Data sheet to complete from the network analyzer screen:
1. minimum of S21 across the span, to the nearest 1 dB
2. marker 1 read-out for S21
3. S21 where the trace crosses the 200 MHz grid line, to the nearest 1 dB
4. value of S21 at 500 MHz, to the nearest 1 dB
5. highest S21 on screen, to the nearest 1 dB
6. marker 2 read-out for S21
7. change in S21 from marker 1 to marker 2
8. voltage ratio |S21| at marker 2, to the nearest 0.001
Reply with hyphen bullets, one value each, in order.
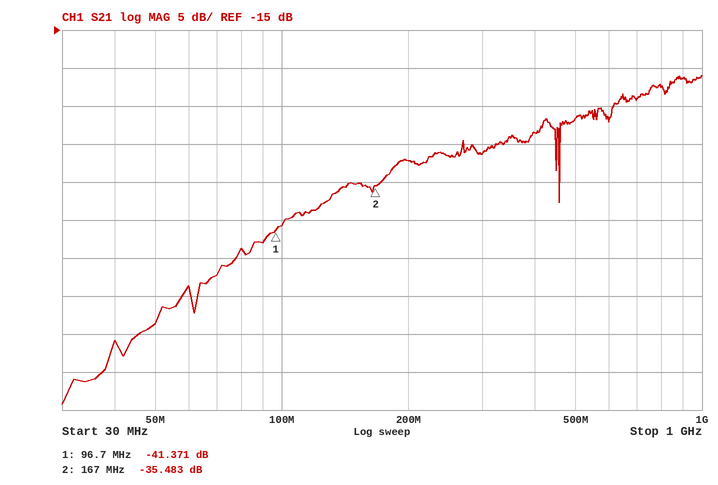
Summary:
- -64 dB
- -41.371 dB
- -32 dB
- -27 dB
- -21 dB
- -35.483 dB
- 5.888 dB
- 0.017
